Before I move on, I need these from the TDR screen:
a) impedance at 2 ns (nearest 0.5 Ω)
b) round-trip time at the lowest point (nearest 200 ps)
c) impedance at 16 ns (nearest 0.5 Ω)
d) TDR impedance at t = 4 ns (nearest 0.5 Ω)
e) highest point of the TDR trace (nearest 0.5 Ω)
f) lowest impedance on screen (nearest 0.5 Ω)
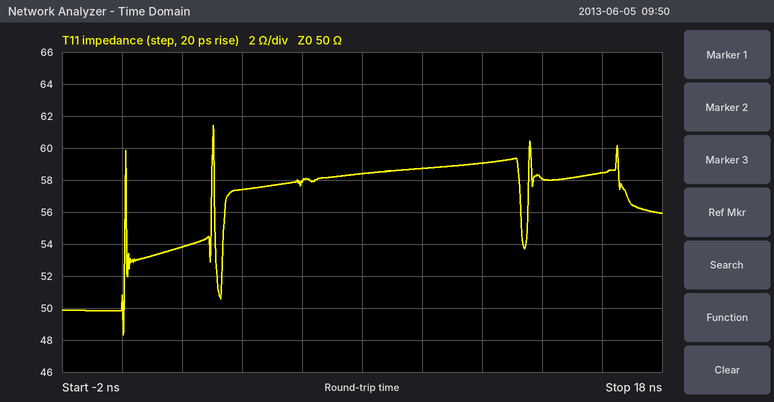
54.0 Ω
0.0 ns
58.5 Ω
57.5 Ω
61.5 Ω
48.5 Ω
